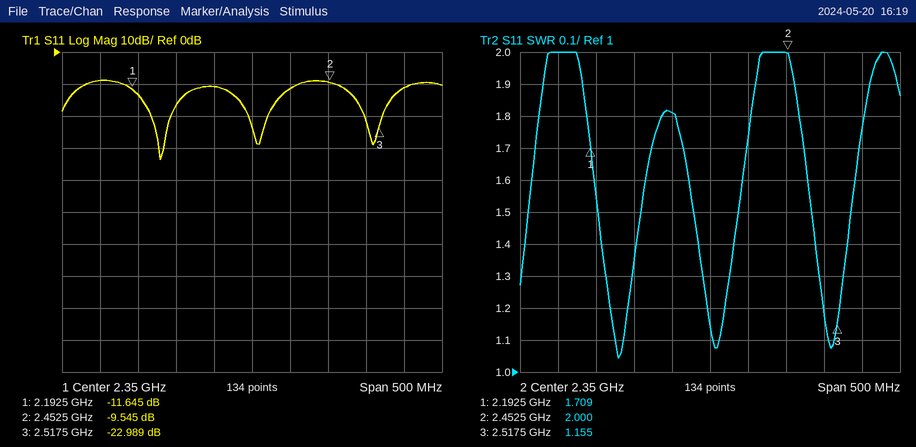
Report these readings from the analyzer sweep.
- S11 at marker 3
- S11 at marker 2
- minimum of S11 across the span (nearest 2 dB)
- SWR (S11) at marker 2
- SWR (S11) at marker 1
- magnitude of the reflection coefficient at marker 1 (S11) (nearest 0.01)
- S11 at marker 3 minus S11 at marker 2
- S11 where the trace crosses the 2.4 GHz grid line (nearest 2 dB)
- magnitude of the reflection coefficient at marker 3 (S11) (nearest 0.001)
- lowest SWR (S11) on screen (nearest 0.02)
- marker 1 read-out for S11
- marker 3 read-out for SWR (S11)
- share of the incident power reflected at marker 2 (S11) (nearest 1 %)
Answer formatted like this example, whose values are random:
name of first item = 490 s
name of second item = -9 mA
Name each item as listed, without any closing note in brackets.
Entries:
S11 at marker 3 = -22.989 dB
S11 at marker 2 = -9.545 dB
minimum of S11 across the span = -34 dB
SWR (S11) at marker 2 = 2.000
SWR (S11) at marker 1 = 1.709
magnitude of the reflection coefficient at marker 1 (S11) = 0.26
S11 at marker 3 minus S11 at marker 2 = -13.444 dB
S11 where the trace crosses the 2.4 GHz grid line = -12 dB
magnitude of the reflection coefficient at marker 3 (S11) = 0.071
lowest SWR (S11) on screen = 1.04
marker 1 read-out for S11 = -11.645 dB
marker 3 read-out for SWR = 1.155
share of the incident power reflected at marker 2 (S11) = 11 %
